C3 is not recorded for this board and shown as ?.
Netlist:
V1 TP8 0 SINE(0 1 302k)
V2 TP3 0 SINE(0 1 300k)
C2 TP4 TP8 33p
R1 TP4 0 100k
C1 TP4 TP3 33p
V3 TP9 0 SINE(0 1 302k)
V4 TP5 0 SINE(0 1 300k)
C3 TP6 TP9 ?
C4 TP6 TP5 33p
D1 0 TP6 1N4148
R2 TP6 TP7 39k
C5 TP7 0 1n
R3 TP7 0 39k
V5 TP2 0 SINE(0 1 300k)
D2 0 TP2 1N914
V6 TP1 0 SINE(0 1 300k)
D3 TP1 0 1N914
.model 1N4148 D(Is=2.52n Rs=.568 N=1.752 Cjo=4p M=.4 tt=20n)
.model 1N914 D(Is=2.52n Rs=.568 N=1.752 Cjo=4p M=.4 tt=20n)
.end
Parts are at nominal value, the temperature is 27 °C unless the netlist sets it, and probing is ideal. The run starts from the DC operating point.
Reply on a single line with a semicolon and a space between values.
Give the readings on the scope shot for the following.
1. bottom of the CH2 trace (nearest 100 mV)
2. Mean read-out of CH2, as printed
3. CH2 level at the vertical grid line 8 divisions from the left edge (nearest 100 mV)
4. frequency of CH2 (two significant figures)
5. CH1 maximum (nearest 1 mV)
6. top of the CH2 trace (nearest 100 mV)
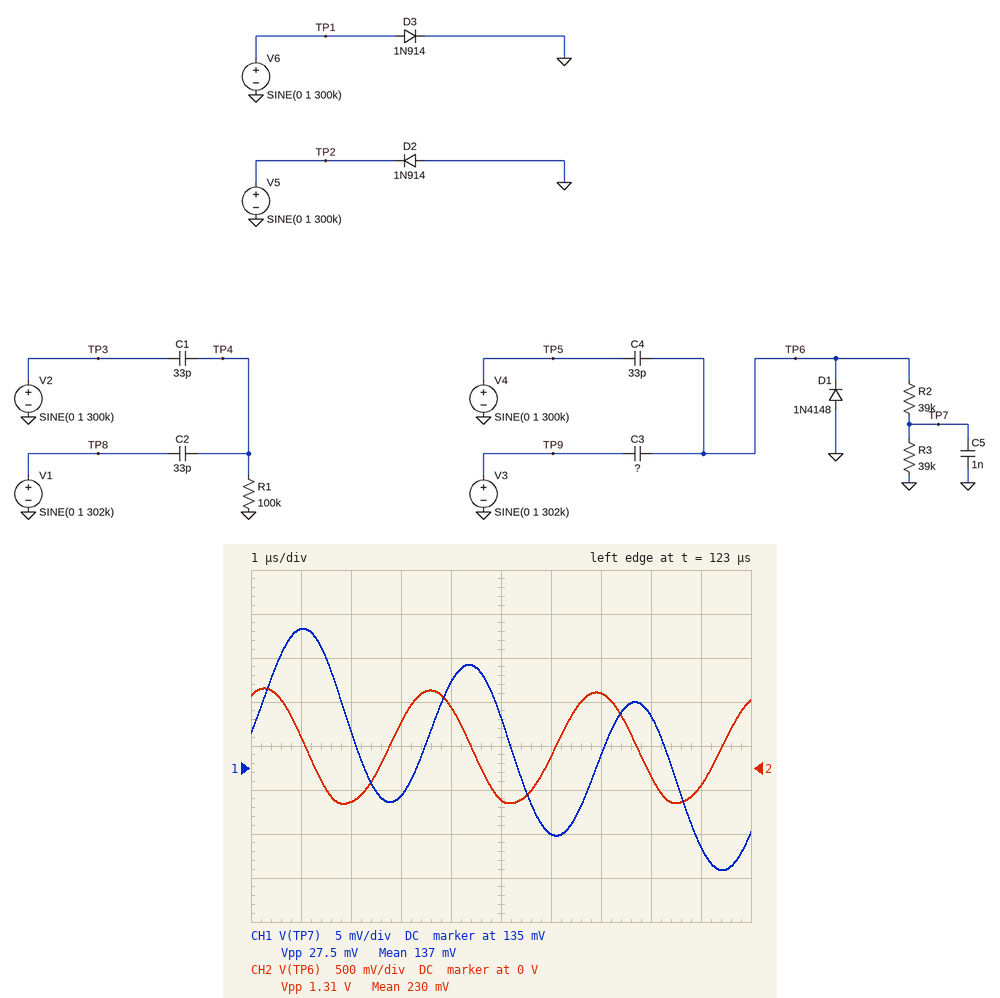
-400 mV; 230 mV; -100 mV; 300 kHz; 151 mV; 900 mV
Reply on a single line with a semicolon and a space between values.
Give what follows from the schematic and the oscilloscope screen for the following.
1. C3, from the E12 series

39 pF
